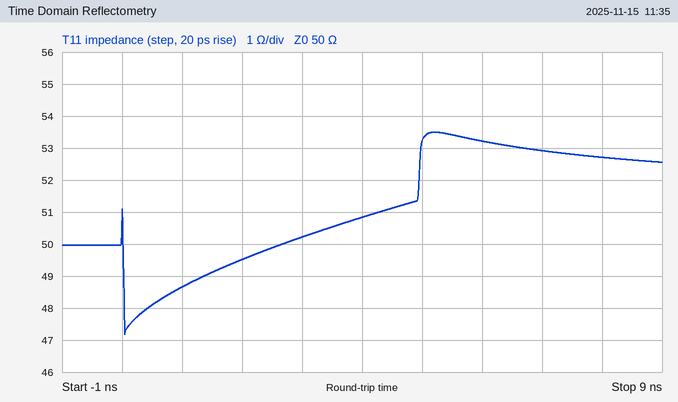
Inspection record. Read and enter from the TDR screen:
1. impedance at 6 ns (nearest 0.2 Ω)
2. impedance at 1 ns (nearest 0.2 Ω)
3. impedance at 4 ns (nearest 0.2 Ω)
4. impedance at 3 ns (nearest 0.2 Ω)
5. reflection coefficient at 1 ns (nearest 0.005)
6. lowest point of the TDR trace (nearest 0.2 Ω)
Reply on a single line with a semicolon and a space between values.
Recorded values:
53.2 Ω; 48.6 Ω; 50.8 Ω; 50.2 Ω; -0.015; 47.2 Ω
